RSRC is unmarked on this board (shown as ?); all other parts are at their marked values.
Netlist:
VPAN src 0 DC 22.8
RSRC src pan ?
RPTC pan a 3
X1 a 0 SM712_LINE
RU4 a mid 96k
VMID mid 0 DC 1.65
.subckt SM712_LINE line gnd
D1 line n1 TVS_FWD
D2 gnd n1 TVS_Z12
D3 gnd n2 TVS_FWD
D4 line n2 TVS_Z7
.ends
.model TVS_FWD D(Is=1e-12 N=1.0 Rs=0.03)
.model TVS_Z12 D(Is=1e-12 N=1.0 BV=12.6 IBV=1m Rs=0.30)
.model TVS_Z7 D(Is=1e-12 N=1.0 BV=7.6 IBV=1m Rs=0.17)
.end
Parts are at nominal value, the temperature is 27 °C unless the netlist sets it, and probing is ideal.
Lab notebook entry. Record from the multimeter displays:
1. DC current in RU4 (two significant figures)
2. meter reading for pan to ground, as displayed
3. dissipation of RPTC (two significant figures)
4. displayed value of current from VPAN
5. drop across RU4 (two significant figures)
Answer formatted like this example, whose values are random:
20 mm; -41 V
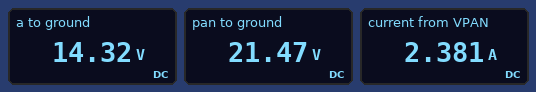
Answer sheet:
130 µA; 21.47 V; 17 W; 2.381 A; 13 V
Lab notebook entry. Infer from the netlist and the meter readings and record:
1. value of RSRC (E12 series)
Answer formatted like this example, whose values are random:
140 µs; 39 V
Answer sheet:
0.56 Ω
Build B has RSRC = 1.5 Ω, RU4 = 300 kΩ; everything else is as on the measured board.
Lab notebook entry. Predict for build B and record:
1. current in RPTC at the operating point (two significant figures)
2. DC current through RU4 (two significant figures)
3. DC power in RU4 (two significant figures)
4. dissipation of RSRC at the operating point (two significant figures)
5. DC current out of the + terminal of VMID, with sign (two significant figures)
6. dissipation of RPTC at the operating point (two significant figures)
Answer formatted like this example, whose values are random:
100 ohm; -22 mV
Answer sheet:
1.9 A; 42 µA; 520 µW; 5.5 W; -42 µA; 11 W
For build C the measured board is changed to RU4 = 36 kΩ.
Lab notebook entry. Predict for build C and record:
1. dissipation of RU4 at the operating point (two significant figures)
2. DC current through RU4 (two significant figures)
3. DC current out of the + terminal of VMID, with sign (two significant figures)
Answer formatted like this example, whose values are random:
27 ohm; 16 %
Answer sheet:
4.5 mW; 350 µA; -350 µA
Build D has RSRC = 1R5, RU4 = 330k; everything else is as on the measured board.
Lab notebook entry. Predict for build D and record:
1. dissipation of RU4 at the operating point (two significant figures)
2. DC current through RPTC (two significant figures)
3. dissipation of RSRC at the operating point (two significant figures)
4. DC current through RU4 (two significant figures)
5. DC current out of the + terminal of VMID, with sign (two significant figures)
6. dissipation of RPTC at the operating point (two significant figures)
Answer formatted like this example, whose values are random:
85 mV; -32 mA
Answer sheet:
470 µW; 1.9 A; 5.5 W; 38 µA; -38 µA; 11 W
